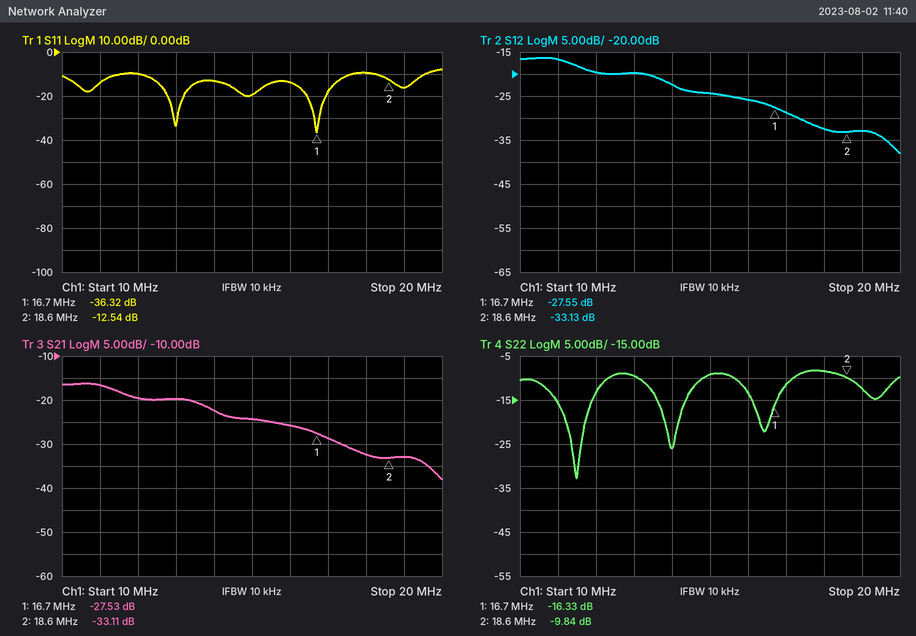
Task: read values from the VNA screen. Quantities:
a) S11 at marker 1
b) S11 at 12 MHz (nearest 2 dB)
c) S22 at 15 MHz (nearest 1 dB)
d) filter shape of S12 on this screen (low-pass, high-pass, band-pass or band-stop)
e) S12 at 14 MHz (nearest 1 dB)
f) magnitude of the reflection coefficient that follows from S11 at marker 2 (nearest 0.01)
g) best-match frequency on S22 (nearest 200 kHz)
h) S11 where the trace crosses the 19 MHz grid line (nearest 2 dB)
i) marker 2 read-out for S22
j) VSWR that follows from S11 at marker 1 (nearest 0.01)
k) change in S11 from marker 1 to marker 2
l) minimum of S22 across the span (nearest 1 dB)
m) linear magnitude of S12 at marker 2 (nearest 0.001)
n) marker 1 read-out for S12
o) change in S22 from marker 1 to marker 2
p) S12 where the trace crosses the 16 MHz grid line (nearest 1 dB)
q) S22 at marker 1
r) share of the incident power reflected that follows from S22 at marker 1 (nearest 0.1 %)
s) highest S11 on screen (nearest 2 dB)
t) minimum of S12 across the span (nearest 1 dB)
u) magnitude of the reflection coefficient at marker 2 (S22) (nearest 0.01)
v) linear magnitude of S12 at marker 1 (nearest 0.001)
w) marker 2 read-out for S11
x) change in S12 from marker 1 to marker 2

-36.32 dB
-10 dB
-9 dB
low-pass
-22 dB
0.24
11.4 MHz
-16 dB
-9.84 dB
1.03
23.78 dB
-33 dB
0.022
-27.55 dB
6.49 dB
-26 dB
-16.33 dB
2.3 %
-8 dB
-38 dB
0.32
0.042
-12.54 dB
-5.58 dB
